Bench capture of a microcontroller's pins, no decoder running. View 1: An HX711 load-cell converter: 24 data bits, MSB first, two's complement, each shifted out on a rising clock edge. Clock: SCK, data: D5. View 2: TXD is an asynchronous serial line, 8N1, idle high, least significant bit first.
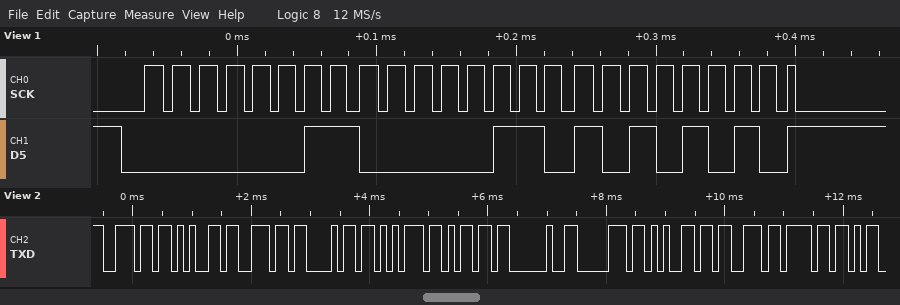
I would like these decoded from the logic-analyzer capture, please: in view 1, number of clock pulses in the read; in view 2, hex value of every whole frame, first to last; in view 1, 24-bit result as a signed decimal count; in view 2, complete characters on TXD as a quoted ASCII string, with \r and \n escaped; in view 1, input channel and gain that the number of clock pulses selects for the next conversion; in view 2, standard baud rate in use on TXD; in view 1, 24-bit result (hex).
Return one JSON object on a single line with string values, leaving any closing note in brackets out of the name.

{"in view 1, number of clock pulses in the read": "25", "in view 2, hex value of every whole frame, first to last": "0x6E 0x65 0x6E 0x68 0x75 0x6D 0x20 0x70 0x65 0x73 0x6F", "in view 1, 24-bit result as a signed decimal count": "198314", "in view 2, complete characters on TXD as a quoted ASCII string, with \\r and \\n escaped": "\"nenhum peso\"", "in view 1, input channel and gain that the number of clock pulses selects for the next conversion": "channel A, gain 128", "in view 2, standard baud rate in use on TXD": "9600 baud", "in view 1, 24-bit result": "0x0306AA"}
